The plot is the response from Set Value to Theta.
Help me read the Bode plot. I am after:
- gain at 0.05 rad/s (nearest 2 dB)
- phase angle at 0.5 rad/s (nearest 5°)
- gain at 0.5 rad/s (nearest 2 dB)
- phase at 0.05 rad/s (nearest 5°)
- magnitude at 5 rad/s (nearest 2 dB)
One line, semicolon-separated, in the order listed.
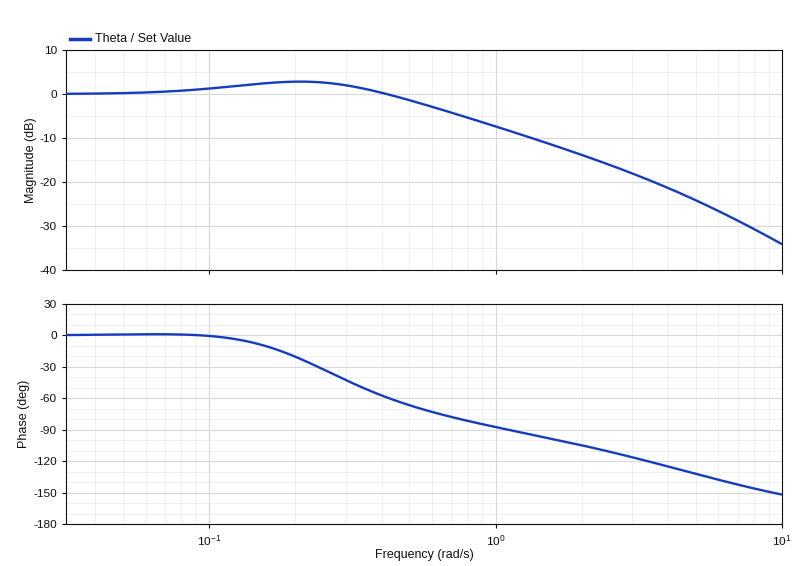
0 dB; -65°; -2 dB; 0°; -24 dB
